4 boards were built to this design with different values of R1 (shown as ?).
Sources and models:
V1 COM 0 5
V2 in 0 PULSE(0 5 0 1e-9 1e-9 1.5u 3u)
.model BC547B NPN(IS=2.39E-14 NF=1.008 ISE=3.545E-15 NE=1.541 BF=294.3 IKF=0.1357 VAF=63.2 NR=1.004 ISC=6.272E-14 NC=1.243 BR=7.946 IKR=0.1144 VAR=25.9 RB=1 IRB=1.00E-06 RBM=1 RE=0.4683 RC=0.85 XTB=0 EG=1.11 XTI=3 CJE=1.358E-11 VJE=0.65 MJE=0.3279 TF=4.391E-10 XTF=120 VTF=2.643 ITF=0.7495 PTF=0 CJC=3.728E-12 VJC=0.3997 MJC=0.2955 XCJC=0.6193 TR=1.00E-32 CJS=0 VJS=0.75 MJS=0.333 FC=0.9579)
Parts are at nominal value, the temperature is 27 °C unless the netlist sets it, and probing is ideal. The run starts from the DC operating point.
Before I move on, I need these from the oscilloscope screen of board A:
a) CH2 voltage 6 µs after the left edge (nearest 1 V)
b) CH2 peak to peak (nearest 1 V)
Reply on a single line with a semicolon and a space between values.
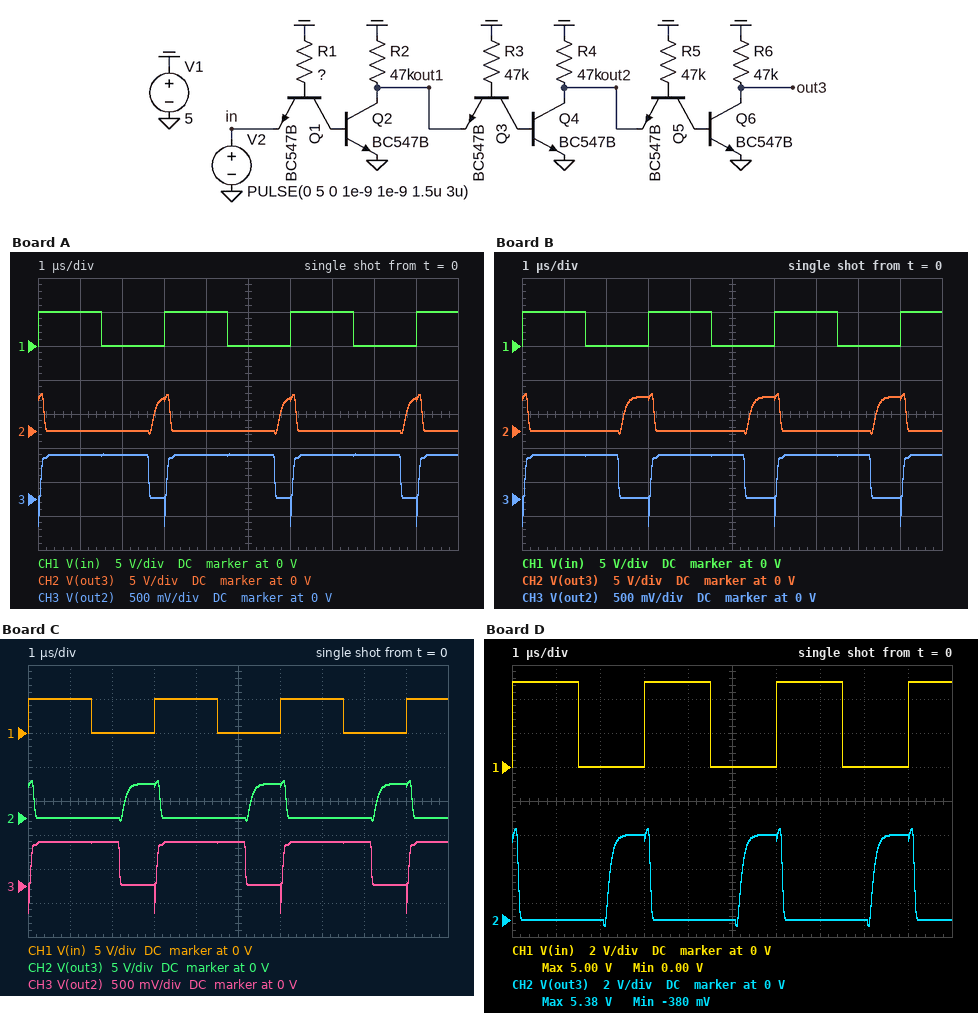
5 V; 6 V
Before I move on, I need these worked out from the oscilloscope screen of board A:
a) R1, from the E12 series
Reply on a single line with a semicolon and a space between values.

150 kΩ
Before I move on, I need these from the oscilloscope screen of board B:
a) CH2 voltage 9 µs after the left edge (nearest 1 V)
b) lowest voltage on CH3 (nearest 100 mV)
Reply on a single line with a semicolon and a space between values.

5 V; -400 mV
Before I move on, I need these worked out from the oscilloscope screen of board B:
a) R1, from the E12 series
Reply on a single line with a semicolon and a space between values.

100 kΩ
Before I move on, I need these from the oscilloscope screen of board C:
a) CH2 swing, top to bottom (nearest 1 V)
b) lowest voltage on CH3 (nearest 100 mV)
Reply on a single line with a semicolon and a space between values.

6 V; -400 mV
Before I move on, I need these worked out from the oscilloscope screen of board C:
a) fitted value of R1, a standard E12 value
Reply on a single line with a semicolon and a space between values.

82 kΩ
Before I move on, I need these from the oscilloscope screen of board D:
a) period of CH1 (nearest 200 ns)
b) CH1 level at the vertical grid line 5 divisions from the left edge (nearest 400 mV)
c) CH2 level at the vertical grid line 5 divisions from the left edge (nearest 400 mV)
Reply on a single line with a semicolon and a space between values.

3.0 µs; 0 V; 0 V
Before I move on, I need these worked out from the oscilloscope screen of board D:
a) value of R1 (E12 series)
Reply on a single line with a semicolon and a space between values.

68 kΩ
